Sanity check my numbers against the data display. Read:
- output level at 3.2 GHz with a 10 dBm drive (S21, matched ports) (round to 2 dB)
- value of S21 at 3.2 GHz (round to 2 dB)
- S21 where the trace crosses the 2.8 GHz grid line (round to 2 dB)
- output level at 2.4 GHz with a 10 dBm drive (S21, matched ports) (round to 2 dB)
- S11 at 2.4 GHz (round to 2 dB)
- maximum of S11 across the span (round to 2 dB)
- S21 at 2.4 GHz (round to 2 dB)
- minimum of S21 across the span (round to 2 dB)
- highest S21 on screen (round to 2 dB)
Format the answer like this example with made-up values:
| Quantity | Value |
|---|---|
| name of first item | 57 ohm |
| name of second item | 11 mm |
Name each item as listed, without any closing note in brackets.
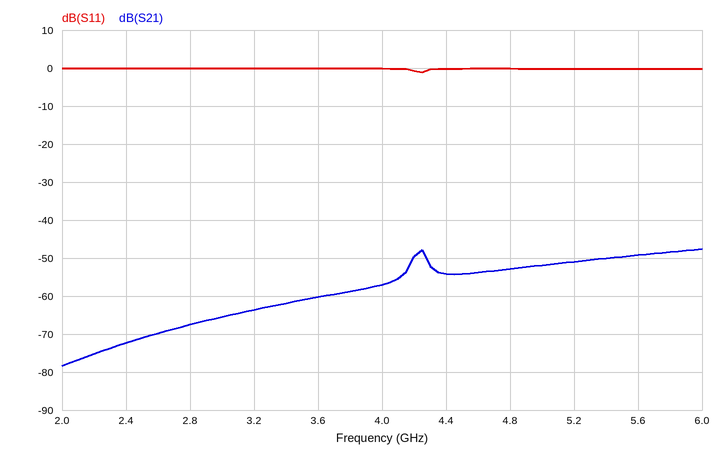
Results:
| Quantity | Value |
|---|---|
| output level at 3.2 GHz with a 10 dBm drive (S21, matched ports) | -54 dBm |
| value of S21 at 3.2 GHz | -64 dB |
| S21 where the trace crosses the 2.8 GHz grid line | -68 dB |
| output level at 2.4 GHz with a 10 dBm drive (S21, matched ports) | -62 dBm |
| S11 at 2.4 GHz | 0 dB |
| maximum of S11 across the span | 0 dB |
| S21 at 2.4 GHz | -72 dB |
| minimum of S21 across the span | -78 dB |
| highest S21 on screen | -48 dB |
